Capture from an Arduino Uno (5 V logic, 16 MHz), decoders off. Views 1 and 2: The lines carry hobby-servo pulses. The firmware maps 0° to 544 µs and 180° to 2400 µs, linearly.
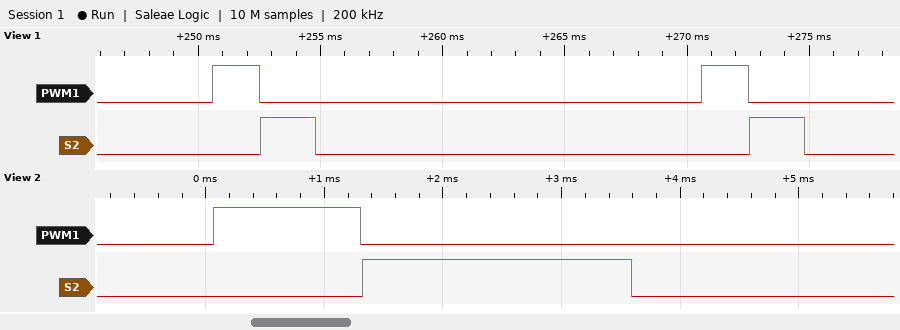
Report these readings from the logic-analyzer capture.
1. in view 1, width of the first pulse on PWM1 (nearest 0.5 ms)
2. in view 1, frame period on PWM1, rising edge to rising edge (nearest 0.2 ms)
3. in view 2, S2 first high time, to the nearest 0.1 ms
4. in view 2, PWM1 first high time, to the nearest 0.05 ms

2.0 ms
20.0 ms
2.3 ms
1.25 ms
